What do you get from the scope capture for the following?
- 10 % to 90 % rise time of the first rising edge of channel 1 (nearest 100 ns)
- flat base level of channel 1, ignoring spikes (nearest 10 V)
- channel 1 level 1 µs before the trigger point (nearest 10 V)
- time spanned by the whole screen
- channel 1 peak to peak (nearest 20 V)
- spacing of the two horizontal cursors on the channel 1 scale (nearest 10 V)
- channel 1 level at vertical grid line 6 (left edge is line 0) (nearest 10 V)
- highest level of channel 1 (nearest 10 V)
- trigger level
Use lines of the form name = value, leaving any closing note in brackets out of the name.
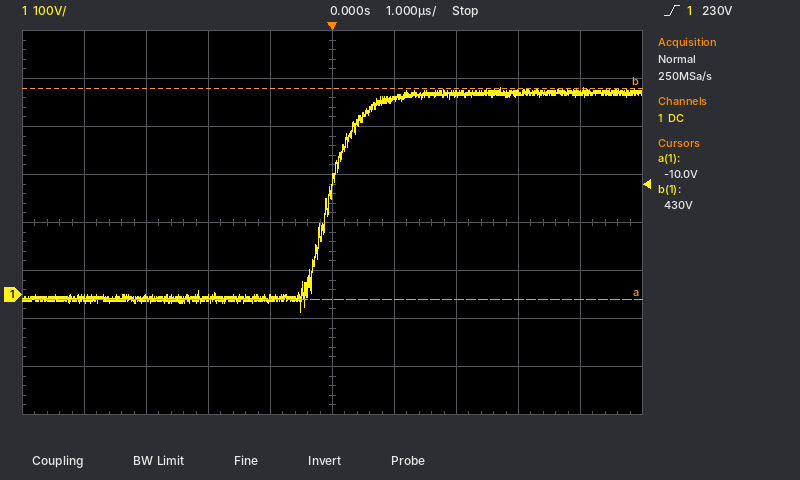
10 % to 90 % rise time of the first rising edge of channel 1 = 900 ns
flat base level of channel 1, ignoring spikes = -10 V
channel 1 level 1 µs before the trigger point = -10 V
time spanned by the whole screen = 10 µs
channel 1 peak to peak = 460 V
spacing of the two horizontal cursors on the channel 1 scale = 440 V
channel 1 level at vertical grid line 6 (left edge is line 0) = 410 V
highest level of channel 1 = 430 V
trigger level = 230 V
